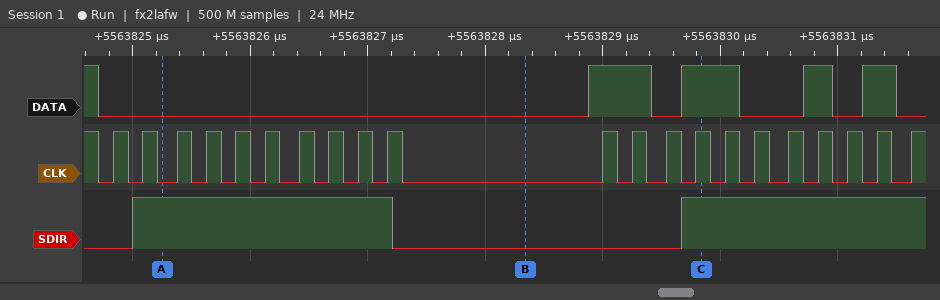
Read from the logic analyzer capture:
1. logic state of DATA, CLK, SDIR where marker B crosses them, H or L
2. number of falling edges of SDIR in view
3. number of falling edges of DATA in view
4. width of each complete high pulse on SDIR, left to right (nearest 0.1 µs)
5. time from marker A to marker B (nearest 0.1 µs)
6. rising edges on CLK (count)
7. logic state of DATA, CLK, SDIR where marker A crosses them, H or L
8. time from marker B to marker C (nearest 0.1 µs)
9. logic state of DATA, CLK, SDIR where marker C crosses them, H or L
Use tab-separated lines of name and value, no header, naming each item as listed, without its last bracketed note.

logic state of DATA, CLK, SDIR where marker B crosses them, H or L	DATA=L, CLK=L, SDIR=L
number of falling edges of SDIR in view	1
number of falling edges of DATA in view	5
width of each complete high pulse on SDIR, left to right	2.2 µs
time from marker A to marker B	3.1 µs
rising edges on CLK	21
logic state of DATA, CLK, SDIR where marker A crosses them, H or L	DATA=L, CLK=L, SDIR=H
time from marker B to marker C	1.5 µs
logic state of DATA, CLK, SDIR where marker C crosses them, H or L	DATA=H, CLK=H, SDIR=H
